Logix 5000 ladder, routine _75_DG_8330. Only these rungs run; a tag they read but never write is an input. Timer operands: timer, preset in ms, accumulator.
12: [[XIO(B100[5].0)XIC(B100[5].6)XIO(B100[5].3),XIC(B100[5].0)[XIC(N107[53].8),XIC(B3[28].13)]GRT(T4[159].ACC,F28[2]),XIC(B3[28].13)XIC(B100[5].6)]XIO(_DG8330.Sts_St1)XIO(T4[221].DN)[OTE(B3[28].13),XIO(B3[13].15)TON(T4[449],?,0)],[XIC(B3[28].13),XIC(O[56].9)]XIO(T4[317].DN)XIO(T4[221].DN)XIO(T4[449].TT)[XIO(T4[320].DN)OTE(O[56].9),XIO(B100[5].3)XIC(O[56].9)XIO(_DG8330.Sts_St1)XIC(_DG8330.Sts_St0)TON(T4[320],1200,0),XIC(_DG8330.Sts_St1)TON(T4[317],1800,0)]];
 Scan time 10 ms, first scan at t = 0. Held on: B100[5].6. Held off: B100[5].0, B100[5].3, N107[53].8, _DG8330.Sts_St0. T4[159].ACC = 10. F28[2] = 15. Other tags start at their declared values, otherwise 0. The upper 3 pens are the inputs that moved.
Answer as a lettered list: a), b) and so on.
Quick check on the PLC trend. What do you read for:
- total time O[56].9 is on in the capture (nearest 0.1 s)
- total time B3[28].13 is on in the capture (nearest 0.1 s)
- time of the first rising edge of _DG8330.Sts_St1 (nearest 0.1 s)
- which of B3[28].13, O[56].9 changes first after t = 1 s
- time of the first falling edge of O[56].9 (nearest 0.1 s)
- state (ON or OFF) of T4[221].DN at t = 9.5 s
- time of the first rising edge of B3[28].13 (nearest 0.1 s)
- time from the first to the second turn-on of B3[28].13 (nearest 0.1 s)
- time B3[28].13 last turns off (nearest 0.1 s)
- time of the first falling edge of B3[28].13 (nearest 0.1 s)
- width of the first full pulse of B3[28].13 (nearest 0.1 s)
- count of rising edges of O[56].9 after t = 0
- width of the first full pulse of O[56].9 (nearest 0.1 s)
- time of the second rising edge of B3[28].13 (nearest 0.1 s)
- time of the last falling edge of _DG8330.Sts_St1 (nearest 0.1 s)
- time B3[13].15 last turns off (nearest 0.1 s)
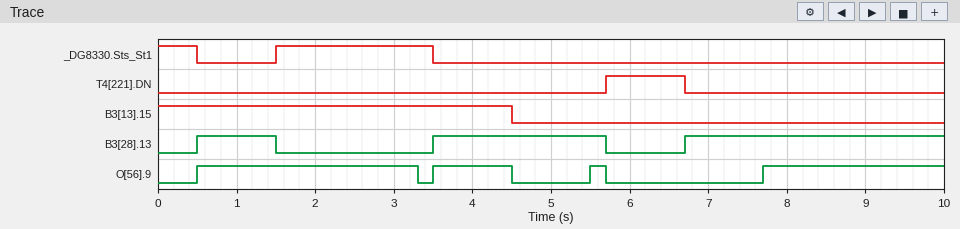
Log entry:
a) 6.3 s
b) 6.5 s
c) 1.5 s
d) B3[28].13
e) 3.3 s
f) OFF
g) 0.5 s
h) 3.0 s
i) 5.7 s
j) 1.5 s
k) 1.0 s
l) 4
m) 2.8 s
n) 3.5 s
o) 3.5 s
p) 4.5 s
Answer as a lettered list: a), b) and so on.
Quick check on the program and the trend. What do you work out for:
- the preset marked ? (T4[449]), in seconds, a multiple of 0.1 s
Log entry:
a) 1.0 s
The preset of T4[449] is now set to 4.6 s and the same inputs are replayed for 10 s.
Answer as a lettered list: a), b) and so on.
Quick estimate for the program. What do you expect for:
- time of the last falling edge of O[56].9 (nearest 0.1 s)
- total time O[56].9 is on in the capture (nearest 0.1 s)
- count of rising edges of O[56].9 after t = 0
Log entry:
a) 4.5 s
b) 3.8 s
c) 2
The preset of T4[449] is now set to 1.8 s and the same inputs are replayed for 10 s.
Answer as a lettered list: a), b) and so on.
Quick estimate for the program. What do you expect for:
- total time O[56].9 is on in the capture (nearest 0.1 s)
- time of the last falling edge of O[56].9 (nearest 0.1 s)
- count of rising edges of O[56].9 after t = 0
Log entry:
a) 5.3 s
b) 4.5 s
c) 3
